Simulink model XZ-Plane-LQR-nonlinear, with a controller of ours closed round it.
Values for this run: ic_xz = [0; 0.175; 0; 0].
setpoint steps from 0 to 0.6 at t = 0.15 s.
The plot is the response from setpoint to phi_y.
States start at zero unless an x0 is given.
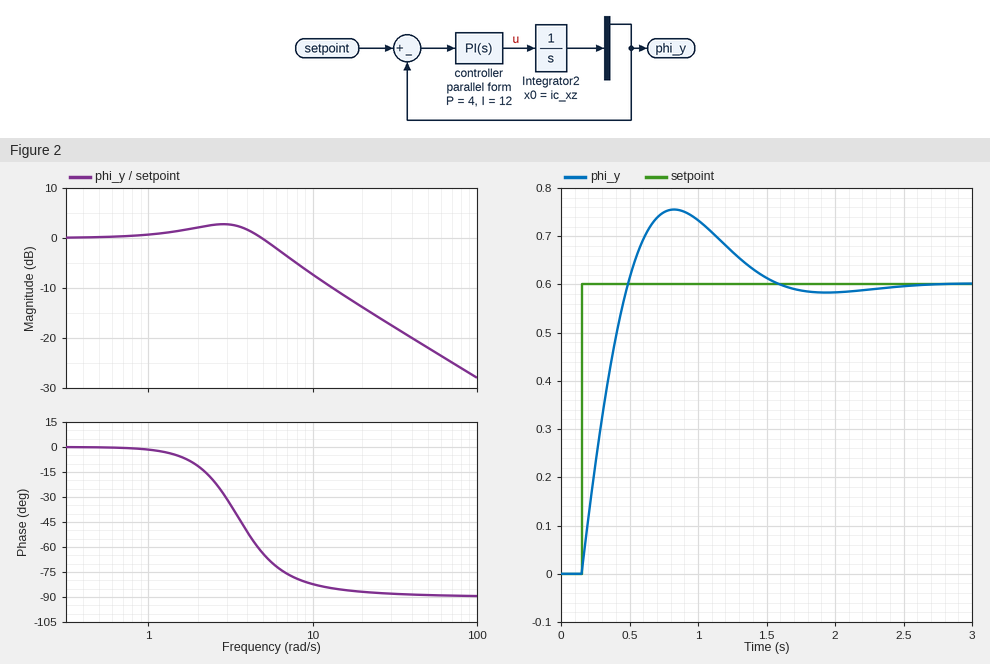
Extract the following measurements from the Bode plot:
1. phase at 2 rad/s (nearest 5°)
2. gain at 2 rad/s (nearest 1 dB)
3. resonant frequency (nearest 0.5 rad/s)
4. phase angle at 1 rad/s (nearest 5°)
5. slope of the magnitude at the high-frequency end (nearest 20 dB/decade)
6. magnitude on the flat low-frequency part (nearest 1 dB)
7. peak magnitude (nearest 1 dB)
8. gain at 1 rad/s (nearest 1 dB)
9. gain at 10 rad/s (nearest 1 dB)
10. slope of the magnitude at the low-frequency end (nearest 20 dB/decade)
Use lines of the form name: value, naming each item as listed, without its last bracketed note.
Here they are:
phase at 2 rad/s: -10°
gain at 2 rad/s: 2 dB
resonant frequency: 3.0 rad/s
phase angle at 1 rad/s: 0°
slope of the magnitude at the high-frequency end: -20 dB/decade
magnitude on the flat low-frequency part: 0 dB
peak magnitude: 3 dB
gain at 1 rad/s: 1 dB
gain at 10 rad/s: -7 dB
slope of the magnitude at the low-frequency end: 0 dB/decade
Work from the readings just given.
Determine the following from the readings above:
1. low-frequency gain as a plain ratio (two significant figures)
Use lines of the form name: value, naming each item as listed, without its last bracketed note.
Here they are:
low-frequency gain as a plain ratio: 1.0
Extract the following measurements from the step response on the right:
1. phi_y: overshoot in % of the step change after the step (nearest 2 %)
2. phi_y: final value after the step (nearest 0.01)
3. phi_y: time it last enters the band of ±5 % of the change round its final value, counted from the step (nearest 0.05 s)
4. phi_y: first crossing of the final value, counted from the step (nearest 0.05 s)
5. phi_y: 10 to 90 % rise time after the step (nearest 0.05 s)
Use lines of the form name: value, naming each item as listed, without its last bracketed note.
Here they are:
phi_y: overshoot in % of the step change after the step: 26 %
phi_y: final value after the step: 0.60
phi_y: time it last enters the band of ±5 % of the change round its final value, counted from the step: 1.25 s
phi_y: first crossing of the final value, counted from the step: 0.35 s
phi_y: 10 to 90 % rise time after the step: 0.25 s
